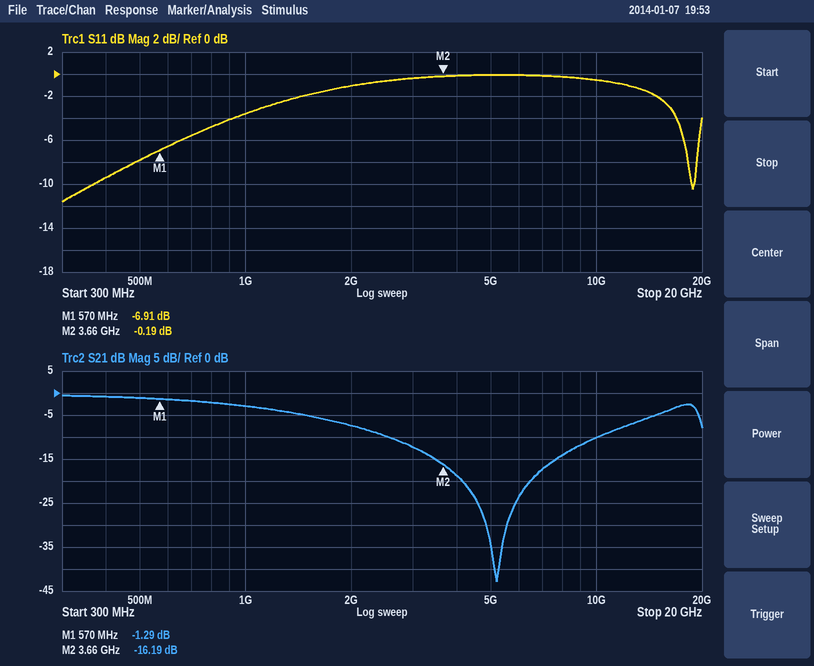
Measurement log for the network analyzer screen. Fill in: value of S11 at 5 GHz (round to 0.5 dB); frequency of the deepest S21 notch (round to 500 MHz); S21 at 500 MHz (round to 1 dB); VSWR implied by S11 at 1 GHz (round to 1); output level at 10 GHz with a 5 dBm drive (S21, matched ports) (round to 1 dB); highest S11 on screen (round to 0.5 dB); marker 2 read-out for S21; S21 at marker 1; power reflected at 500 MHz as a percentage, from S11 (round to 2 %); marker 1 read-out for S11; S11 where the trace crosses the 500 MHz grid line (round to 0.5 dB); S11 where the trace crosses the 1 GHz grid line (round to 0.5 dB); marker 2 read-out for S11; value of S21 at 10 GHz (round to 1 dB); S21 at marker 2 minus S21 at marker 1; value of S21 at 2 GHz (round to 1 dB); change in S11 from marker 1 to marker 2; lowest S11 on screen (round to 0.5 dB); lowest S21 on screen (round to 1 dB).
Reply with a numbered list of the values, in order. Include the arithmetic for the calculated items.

1. 0.0 dB
2. 5.0 GHz
3. -1 dB
4. |Γ| = 10^(-3.5/20) = 0.6683; VSWR = (1 + 0.6683)/(1 − 0.6683) ≈ 5
5. 5 dBm + (-10 dB) = -5 dBm
6. 0.0 dB
7. -16.19 dB
8. -1.29 dB
9. 10^(-8/10) ≈ 16 %
10. -6.91 dB
11. -8.0 dB
12. -3.5 dB
13. -0.19 dB
14. -10 dB
15. -16.19 − (-1.29) = -14.90 dB
16. -7 dB
17. -0.19 − (-6.91) = 6.72 dB
18. -11.5 dB
19. -43 dB
